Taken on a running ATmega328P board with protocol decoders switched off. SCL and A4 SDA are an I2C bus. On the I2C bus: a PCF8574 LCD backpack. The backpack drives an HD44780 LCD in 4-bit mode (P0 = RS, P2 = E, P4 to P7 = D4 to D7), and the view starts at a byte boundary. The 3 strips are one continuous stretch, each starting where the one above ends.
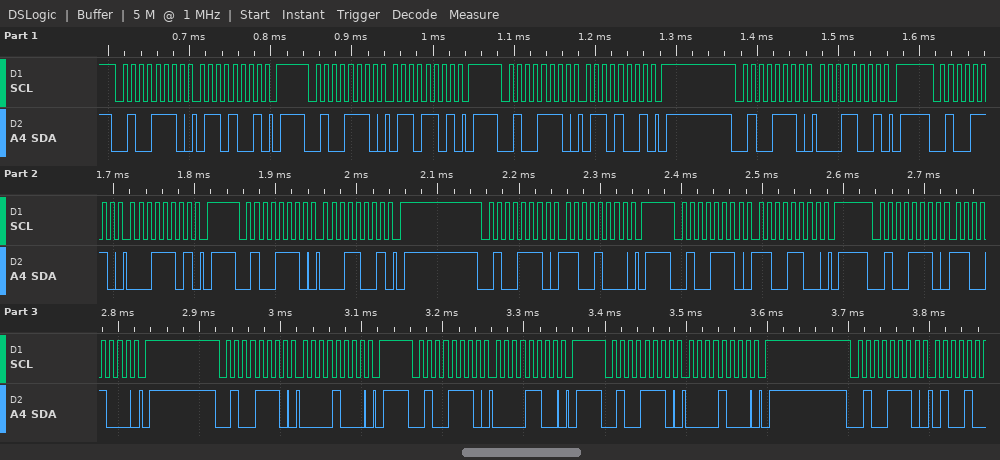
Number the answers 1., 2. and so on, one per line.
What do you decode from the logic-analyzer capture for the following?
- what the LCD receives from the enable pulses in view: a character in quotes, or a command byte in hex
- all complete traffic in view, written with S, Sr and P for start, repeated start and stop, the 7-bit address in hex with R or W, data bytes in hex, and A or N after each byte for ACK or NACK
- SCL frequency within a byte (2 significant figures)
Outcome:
1. 'a' 0xC0
2. S 27W A 69 A P S 27W A 6D A P S 27W A 69 A P S 27W A 19 A P S 27W A 1D A P S 27W A 19 A P S 27W A C8 A P S 27W A CC A P S 27W A C8 A P S 27W A 08 A P S 27W A 0C A P S 27W A 08 A P S 27W A
3. 100 kHz
